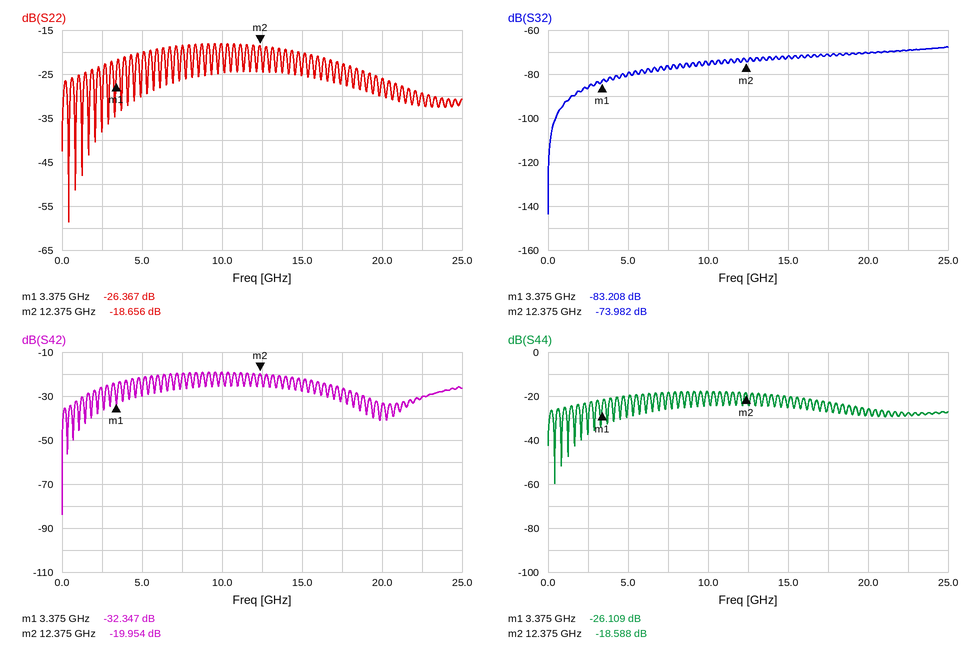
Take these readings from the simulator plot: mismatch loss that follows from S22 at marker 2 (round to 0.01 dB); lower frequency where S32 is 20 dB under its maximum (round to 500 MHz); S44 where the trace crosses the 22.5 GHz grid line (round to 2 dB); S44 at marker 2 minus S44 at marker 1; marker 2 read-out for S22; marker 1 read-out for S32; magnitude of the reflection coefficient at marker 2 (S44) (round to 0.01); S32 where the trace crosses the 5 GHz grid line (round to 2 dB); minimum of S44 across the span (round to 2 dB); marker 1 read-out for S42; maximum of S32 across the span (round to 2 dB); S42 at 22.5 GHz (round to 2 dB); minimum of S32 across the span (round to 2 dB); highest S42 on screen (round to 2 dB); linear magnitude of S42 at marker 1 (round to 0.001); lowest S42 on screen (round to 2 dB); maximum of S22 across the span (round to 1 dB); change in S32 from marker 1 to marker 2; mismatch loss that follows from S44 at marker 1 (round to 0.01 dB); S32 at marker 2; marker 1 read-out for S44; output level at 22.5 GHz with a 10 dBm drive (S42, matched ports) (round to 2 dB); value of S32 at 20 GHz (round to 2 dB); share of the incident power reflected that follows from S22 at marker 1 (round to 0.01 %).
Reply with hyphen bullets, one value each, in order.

- 0.06 dB
- 2.0 GHz
- -28 dB
- 7.521 dB
- -18.656 dB
- -83.208 dB
- 0.12
- -80 dB
- -60 dB
- -32.347 dB
- -68 dB
- -30 dB
- -144 dB
- -20 dB
- 0.024
- -84 dB
- -18 dB
- 9.226 dB
- 0.01 dB
- -73.982 dB
- -26.109 dB
- -20 dBm
- -70 dB
- 0.23 %
